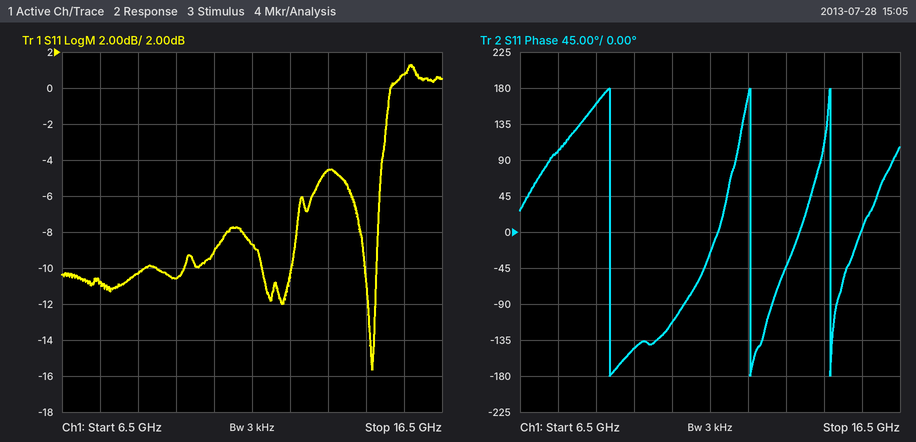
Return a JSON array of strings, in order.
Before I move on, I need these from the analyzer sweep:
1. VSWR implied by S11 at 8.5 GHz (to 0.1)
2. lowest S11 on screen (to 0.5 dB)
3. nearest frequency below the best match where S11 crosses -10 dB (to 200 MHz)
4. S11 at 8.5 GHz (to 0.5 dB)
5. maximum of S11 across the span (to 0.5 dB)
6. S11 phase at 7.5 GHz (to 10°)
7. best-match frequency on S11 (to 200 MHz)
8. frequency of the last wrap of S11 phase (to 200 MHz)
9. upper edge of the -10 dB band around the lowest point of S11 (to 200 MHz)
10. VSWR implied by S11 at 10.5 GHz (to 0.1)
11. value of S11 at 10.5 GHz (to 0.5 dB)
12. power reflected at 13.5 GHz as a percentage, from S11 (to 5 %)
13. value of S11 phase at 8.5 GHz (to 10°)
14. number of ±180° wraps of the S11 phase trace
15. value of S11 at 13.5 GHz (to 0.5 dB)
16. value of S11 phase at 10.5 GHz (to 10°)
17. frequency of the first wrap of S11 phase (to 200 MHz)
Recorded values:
["1.9", "-15.5 dB", "14.4 GHz", "-10.5 dB", "1.5 dB", "100°", "14.6 GHz", "14.6 GHz", "14.8 GHz", "2.1", "-9.0 dB", "35 %", "160°", "3", "-4.5 dB", "-110°", "8.8 GHz"]
